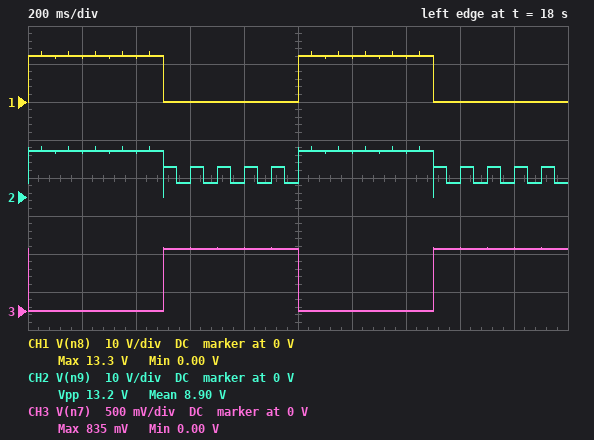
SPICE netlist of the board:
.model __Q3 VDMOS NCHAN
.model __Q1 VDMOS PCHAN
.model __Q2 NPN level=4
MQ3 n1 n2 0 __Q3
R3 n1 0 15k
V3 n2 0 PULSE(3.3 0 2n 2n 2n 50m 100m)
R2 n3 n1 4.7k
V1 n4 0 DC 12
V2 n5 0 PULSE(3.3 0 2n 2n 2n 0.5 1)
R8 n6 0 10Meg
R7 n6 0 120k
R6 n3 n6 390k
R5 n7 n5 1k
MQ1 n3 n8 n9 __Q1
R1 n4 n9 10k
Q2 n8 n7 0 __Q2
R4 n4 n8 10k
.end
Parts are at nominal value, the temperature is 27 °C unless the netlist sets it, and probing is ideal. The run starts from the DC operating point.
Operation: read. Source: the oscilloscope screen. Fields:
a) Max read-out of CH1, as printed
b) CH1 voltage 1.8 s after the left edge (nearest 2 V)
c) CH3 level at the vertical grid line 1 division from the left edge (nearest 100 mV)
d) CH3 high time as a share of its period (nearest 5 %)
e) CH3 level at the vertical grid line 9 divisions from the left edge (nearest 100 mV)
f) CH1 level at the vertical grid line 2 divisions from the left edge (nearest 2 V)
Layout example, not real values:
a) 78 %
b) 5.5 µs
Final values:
a) 13.3 V
b) 0 V
c) 0 V
d) 50 %
e) 800 mV
f) 12 V
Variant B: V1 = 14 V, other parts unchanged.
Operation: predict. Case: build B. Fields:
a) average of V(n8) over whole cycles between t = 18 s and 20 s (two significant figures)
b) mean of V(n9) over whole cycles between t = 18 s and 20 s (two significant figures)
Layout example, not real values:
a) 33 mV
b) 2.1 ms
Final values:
a) 7.0 V
b) 10 V
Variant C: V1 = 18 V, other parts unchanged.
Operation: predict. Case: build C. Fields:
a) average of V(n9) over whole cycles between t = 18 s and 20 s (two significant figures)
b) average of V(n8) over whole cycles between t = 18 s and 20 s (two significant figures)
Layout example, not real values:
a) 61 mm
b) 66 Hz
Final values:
a) 13 V
b) 9.0 V
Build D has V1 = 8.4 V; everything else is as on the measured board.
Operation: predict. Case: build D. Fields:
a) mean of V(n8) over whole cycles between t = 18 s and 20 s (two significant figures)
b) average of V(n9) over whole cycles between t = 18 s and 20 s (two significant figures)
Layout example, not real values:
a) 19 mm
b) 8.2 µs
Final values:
a) 4.2 V
b) 6.3 V
